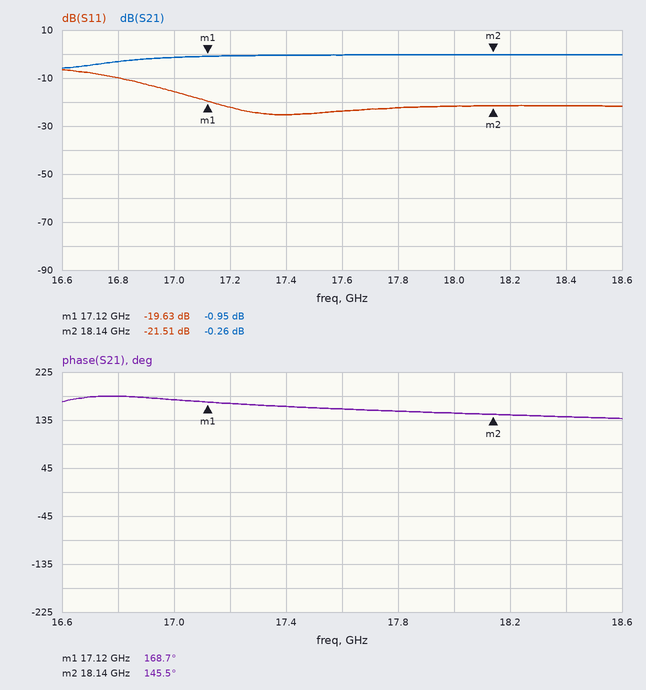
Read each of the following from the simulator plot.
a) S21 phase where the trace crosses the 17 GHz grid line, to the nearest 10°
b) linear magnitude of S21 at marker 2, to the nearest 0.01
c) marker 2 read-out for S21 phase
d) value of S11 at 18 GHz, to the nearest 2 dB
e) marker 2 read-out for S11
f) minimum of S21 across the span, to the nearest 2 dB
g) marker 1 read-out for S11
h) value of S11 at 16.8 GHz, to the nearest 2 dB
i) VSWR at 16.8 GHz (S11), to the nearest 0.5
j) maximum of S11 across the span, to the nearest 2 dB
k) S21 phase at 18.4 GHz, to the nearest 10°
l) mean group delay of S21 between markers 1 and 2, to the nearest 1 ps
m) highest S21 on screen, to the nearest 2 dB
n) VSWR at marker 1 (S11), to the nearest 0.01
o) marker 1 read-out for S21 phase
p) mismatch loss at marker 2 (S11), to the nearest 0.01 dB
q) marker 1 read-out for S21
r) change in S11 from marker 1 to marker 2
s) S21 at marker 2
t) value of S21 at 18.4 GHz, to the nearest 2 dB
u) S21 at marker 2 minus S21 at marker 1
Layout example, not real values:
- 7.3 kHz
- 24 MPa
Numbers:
- 170°
- 0.97
- 145.5°
- -22 dB
- -21.51 dB
- -6 dB
- -19.63 dB
- -10 dB
- 2.0
- -6 dB
- 140°
- 63 ps
- 0 dB
- 1.23
- 168.7°
- 0.03 dB
- -0.95 dB
- -1.88 dB
- -0.26 dB
- 0 dB
- 0.69 dB
